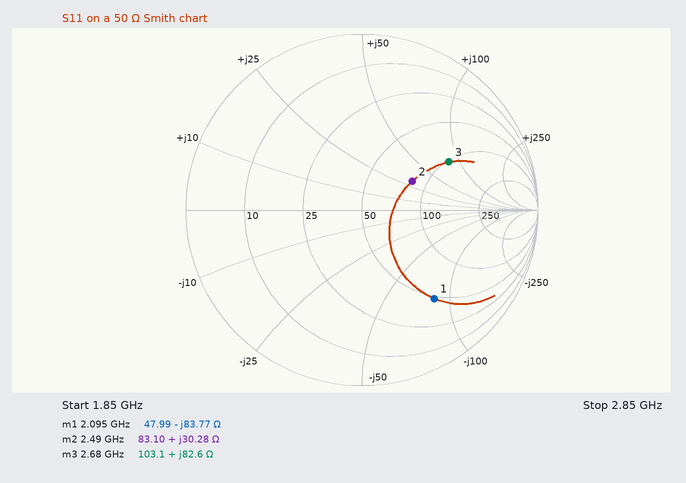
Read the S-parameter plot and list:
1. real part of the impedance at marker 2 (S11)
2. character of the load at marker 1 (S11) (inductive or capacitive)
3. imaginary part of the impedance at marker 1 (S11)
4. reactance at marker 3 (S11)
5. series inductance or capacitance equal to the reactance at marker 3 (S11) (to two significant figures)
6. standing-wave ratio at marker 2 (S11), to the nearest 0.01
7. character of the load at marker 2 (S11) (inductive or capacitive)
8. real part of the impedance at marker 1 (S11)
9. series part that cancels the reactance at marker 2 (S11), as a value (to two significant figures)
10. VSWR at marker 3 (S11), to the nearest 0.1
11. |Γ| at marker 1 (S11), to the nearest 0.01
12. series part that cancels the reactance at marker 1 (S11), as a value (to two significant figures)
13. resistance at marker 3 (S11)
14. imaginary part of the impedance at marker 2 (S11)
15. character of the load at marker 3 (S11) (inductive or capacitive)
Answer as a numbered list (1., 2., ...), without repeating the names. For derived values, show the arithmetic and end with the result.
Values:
1. 83.10 Ω
2. capacitive
3. -83.77 Ω
4. +82.6 Ω
5. L = 82.6 Ω/(2π × 2.68 GHz) ≈ 4.9 nH
6. 1.98
7. inductive
8. 47.99 Ω
9. C = 1/(2π × 2.49 GHz × 30.28 Ω) ≈ 2.1 pF
10. 3.6
11. 0.65
12. L = 83.77 Ω/(2π × 2.095 GHz) ≈ 6.4 nH
13. 103.1 Ω
14. +30.28 Ω
15. inductive
